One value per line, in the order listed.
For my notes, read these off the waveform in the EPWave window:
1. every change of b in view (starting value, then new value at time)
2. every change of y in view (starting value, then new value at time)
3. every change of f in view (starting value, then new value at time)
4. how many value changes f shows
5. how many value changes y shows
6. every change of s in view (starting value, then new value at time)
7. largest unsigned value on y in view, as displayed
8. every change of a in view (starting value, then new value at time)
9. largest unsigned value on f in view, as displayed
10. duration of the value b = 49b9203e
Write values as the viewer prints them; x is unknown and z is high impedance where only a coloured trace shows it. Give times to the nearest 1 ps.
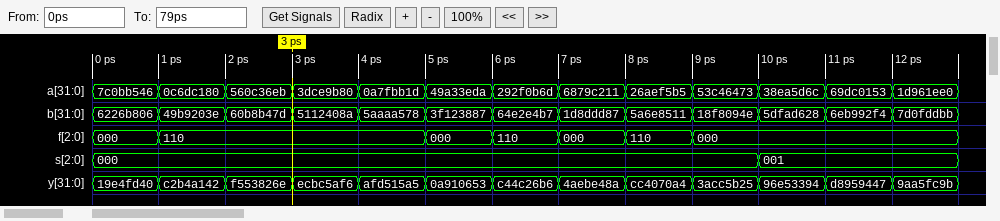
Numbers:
6226b806, 49b9203e at 1 ps, 60b8b47d at 2 ps, 5112408a at 3 ps, 5aaaa578 at 4 ps, 3f123887 at 5 ps, 64e2e4b7 at 6 ps, 1d8ddd87 at 7 ps, 5a6e8511 at 8 ps, 18f8094e at 9 ps, 5dfad628 at 10 ps, 6eb992f4 at 11 ps, 7d0fddbb at 12 ps
19e4fd40, c2b4a142 at 1 ps, f553826e at 2 ps, ecbc5af6 at 3 ps, afd515a5 at 4 ps, 0a910653 at 5 ps, c44c26b6 at 6 ps, 4aebe48a at 7 ps, cc4070a4 at 8 ps, 3acc5b25 at 9 ps, 96e53394 at 10 ps, d8959447 at 11 ps, 9aa5fc9b at 12 ps
000, 110 at 1 ps, 000 at 5 ps, 110 at 6 ps, 000 at 7 ps, 110 at 8 ps, 000 at 9 ps
6
12
000, 001 at 10 ps
f553826e
7c0bb546, 0c6dc180 at 1 ps, 560c36eb at 2 ps, 3dce9b80 at 3 ps, 0a7fbb1d at 4 ps, 49a33eda at 5 ps, 292f0b6d at 6 ps, 6879c211 at 7 ps, 26aef5b5 at 8 ps, 53c46473 at 9 ps, 38ea5d6c at 10 ps, 69dc0153 at 11 ps, 1d961ee0 at 12 ps
110
1 ps
